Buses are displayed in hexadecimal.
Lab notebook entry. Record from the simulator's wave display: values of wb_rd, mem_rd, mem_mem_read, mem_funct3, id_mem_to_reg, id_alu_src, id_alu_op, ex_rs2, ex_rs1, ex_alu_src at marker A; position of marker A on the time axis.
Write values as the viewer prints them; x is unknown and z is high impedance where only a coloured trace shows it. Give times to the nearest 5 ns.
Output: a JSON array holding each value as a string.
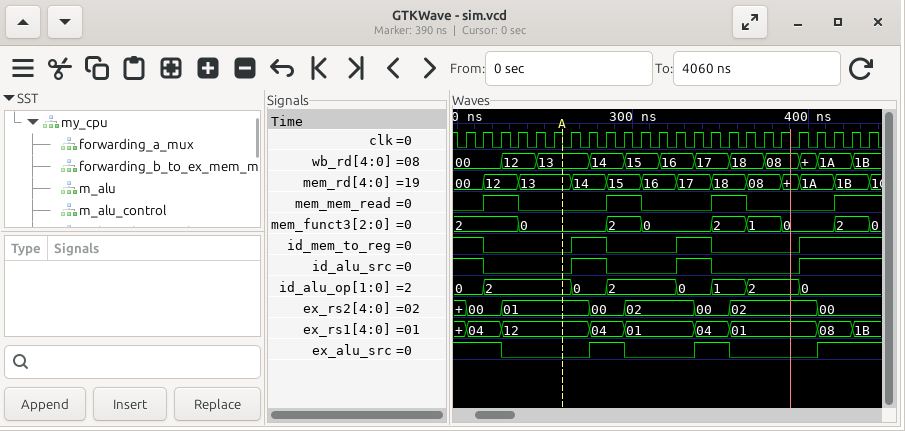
["wb_rd=13, mem_rd=13, mem_mem_read=0, mem_funct3=0, id_mem_to_reg=0, id_alu_src=0, id_alu_op=2, ex_rs2=01, ex_rs1=12, ex_alu_src=0", "260 ns"]
